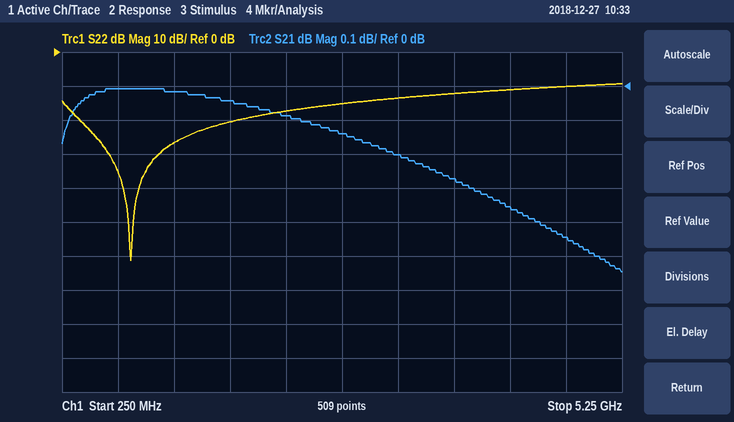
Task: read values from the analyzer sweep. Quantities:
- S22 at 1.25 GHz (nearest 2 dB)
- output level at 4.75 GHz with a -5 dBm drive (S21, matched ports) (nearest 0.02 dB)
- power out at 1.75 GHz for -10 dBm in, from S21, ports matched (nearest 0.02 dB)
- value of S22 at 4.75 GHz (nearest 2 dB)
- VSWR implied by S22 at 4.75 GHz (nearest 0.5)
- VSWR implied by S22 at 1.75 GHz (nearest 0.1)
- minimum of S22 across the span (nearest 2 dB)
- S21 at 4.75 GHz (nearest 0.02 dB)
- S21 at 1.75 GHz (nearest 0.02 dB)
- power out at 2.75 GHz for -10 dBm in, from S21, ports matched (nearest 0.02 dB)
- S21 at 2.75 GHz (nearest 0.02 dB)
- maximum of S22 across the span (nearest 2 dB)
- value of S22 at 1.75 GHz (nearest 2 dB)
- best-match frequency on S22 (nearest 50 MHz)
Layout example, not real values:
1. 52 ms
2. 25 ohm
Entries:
1. -26 dB
2. -5.44 dBm
3. -10.04 dBm
4. -10 dB
5. 2.0
6. 1.2
7. -62 dB
8. -0.44 dB
9. -0.04 dB
10. -10.14 dBm
11. -0.14 dB
12. -10 dB
13. -20 dB
14. 850 MHz
